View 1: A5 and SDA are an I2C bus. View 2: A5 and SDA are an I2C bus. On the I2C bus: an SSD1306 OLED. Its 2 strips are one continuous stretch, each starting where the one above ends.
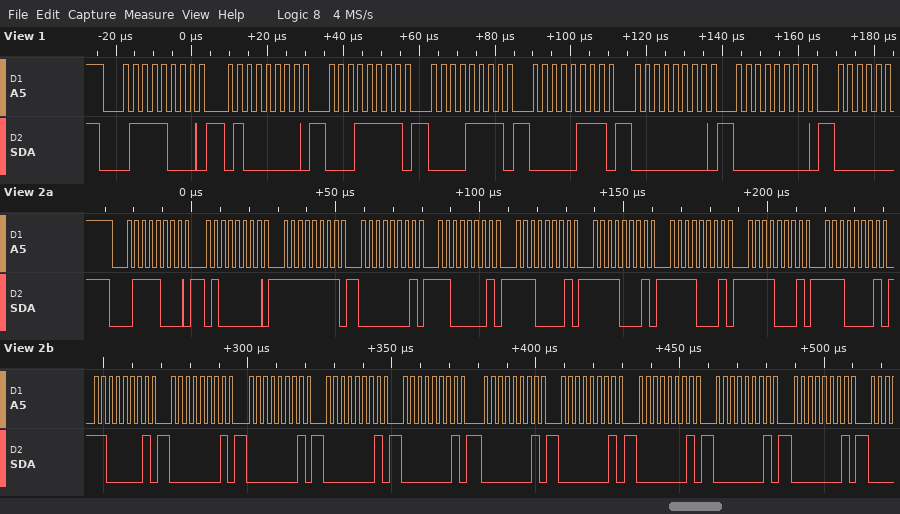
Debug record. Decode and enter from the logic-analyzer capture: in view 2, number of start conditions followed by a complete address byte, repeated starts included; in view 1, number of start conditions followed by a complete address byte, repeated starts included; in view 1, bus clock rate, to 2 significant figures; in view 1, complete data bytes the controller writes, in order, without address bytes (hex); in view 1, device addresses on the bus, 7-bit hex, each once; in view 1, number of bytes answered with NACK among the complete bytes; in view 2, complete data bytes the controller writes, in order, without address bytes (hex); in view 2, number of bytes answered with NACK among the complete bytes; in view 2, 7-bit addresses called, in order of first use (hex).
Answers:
1
1
400 kHz
40 1F 0F 07 00 00
0x3C
0
40 FF 01 C1 E1 F1 F1 F1 E1 C1 01 01 01 01 01 01 01 01 01
0
0x3C
